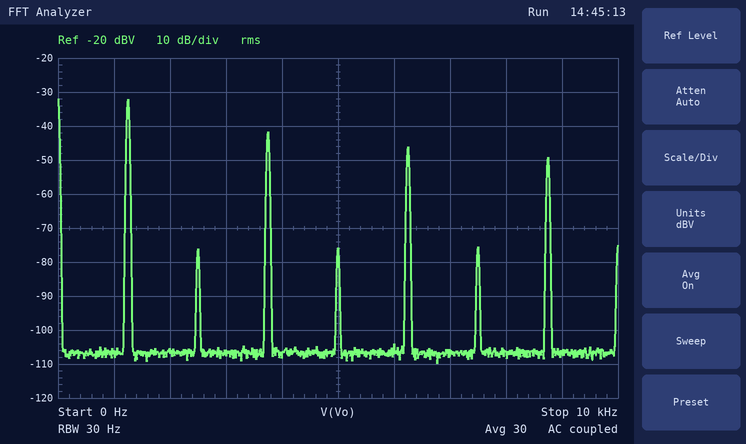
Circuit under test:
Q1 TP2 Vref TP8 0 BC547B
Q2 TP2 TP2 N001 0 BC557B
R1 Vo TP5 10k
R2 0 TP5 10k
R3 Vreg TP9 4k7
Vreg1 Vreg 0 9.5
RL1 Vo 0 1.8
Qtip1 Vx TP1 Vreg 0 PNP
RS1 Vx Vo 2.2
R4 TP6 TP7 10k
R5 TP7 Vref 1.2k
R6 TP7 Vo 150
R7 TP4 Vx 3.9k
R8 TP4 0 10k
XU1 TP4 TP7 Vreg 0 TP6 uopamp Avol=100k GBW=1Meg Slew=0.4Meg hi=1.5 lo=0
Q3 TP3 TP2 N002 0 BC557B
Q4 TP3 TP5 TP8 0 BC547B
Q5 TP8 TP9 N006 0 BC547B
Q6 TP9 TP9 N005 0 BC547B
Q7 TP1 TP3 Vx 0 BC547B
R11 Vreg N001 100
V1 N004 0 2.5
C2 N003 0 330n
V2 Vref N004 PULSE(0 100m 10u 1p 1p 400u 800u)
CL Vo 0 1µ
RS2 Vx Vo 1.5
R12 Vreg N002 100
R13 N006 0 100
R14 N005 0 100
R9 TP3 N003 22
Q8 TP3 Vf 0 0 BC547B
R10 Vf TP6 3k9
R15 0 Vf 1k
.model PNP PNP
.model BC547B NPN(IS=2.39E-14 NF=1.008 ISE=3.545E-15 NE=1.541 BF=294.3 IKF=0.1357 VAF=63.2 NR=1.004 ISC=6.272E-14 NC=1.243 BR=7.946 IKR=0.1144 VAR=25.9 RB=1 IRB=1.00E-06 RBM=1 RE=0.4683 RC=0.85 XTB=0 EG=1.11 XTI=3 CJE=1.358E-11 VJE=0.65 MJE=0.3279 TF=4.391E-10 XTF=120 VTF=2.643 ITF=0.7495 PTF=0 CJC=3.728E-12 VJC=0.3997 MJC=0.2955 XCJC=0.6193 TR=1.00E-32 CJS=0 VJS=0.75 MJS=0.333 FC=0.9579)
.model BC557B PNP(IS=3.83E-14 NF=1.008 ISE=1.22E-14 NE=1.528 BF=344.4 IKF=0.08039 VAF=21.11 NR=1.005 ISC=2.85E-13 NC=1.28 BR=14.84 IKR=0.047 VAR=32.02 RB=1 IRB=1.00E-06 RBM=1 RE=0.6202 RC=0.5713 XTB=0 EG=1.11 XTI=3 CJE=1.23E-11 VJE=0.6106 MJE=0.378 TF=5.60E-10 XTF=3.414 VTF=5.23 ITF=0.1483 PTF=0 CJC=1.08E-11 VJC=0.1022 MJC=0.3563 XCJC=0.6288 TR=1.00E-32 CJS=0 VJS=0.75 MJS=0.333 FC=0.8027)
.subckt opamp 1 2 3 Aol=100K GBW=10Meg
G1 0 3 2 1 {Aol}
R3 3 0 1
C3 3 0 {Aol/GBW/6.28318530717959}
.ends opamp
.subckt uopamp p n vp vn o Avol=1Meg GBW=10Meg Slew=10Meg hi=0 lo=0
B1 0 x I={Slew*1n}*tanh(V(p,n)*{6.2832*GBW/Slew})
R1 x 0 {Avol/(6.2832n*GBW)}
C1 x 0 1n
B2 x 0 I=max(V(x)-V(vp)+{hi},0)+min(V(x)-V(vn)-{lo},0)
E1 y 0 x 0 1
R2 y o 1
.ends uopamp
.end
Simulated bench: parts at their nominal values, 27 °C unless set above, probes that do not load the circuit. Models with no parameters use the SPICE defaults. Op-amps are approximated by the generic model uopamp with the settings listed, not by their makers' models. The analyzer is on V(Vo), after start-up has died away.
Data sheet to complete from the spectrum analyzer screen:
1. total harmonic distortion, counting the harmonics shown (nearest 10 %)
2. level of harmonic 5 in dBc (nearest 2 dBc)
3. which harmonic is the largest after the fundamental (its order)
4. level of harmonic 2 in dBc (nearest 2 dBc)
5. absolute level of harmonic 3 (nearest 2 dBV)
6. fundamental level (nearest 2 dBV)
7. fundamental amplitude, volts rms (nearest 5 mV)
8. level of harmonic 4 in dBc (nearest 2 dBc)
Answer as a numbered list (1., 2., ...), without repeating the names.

1. 40 %
2. -14 dBc
3. 3
4. -44 dBc
5. -42 dBV
6. -32 dBV
7. 25 mV
8. -44 dBc
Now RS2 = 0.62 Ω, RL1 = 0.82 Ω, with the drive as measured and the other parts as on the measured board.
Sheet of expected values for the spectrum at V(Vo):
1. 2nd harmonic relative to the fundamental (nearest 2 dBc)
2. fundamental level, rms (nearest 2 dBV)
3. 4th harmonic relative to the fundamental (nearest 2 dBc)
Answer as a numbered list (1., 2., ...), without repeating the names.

1. -46 dBc
2. -34 dBV
3. -46 dBc
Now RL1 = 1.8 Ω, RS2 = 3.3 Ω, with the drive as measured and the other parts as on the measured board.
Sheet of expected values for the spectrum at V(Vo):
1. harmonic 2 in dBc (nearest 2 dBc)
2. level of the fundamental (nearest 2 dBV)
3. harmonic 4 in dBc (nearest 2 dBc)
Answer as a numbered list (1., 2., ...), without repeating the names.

1. -52 dBc
2. -38 dBV
3. -52 dBc
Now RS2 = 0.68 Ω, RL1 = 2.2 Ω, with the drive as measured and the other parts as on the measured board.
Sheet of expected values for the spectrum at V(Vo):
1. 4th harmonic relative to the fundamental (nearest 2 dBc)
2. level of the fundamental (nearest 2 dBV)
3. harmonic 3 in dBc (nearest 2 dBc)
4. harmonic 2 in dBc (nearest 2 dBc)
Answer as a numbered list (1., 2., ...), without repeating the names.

1. -48 dBc
2. -22 dBV
3. -12 dBc
4. -46 dBc
